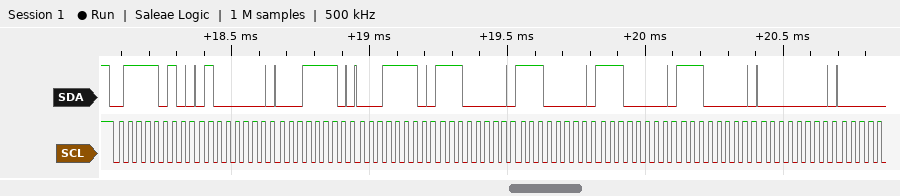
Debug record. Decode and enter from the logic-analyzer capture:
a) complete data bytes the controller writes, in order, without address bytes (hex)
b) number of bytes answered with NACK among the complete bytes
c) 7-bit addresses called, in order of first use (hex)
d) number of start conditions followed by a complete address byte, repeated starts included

40 1E 1E E0 E0 E0 E0 00
0
0x3D
1
